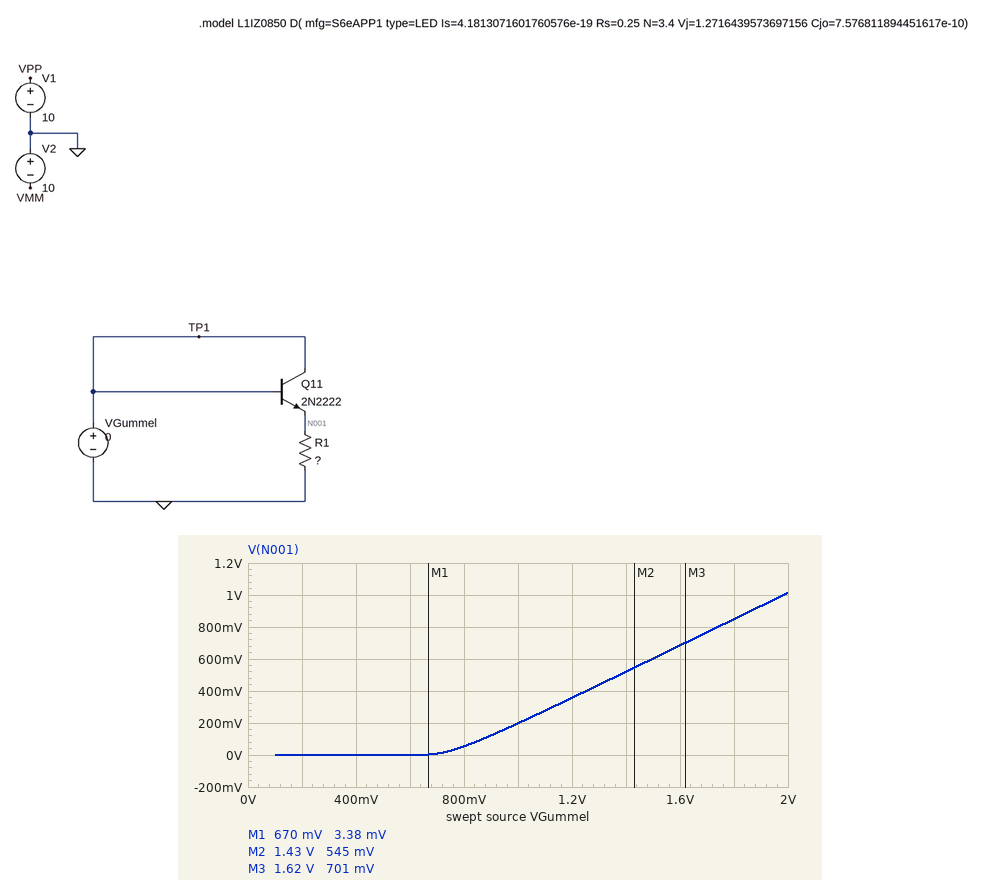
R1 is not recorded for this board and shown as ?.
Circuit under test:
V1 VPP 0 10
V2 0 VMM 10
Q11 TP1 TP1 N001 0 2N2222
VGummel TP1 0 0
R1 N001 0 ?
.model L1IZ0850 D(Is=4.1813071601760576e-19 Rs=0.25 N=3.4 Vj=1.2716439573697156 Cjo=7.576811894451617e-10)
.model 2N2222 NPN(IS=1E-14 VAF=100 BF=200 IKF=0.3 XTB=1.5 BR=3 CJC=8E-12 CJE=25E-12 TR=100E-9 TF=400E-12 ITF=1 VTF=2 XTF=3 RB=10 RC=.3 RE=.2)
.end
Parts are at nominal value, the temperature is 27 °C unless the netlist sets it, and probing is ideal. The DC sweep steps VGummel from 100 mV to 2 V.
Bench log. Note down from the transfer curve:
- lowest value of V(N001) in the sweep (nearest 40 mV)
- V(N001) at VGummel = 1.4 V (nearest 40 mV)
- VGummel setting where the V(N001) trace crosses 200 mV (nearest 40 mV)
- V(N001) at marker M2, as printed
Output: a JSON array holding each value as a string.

["0 V", "520 mV", "1.00 V", "545 mV"]
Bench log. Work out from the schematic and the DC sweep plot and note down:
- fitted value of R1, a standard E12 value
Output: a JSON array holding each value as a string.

["2.2 Ω"]
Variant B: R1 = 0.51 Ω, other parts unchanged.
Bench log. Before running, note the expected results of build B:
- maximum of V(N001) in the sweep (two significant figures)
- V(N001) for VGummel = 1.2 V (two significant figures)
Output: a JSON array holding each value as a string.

["600 mV", "220 mV"]
